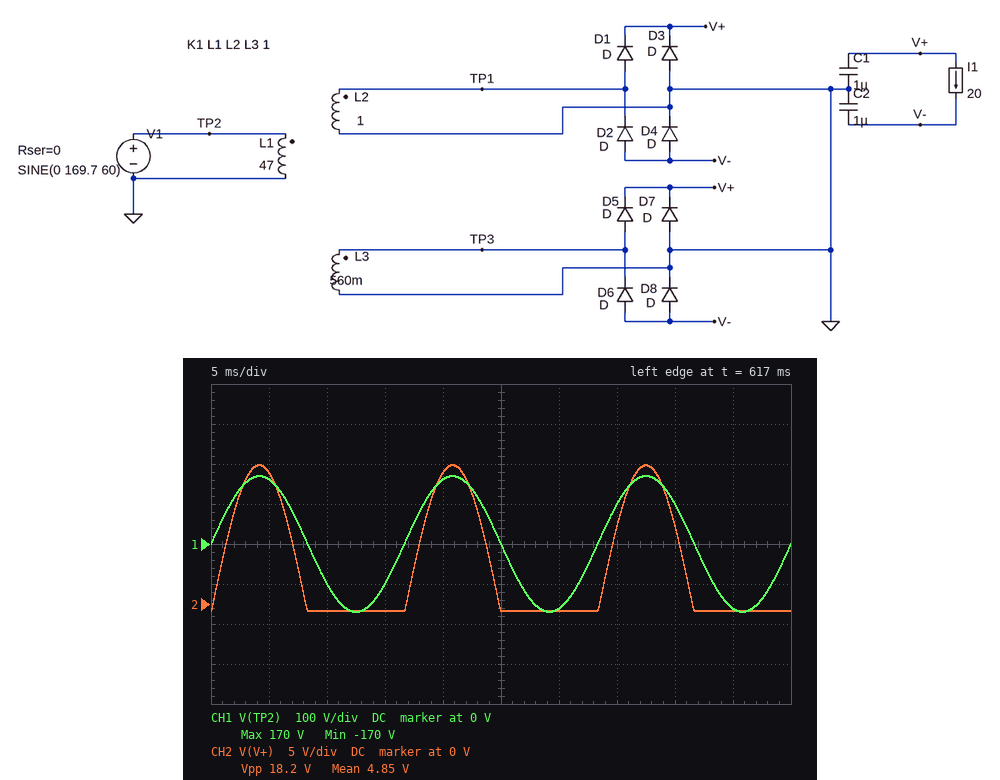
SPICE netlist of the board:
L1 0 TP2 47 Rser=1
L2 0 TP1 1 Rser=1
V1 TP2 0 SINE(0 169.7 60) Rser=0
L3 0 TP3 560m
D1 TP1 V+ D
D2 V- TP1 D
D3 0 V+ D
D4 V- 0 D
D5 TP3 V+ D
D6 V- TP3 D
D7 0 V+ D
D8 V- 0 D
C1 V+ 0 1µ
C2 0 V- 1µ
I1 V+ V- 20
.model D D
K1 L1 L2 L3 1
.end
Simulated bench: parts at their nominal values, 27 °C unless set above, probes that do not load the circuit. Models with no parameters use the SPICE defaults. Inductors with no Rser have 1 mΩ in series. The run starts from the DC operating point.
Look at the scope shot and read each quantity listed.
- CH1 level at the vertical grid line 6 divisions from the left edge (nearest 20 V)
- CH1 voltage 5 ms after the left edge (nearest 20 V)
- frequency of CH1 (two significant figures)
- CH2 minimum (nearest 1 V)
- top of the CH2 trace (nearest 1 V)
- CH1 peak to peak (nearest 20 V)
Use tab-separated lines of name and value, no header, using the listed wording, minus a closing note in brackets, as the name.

CH1 level at the vertical grid line 6 divisions from the left edge	-160 V
CH1 voltage 5 ms after the left edge	160 V
frequency of CH1	60 Hz
CH2 minimum	-1 V
top of the CH2 trace	17 V
CH1 peak to peak	340 V
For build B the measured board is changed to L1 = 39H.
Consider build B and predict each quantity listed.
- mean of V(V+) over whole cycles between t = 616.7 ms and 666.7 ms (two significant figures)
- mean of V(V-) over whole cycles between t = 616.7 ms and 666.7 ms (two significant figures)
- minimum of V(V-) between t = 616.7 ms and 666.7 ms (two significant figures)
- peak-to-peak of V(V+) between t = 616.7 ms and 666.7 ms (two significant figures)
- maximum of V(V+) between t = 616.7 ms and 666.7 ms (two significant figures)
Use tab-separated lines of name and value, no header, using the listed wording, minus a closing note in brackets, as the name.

mean of V(V+) over whole cycles between t = 616.7 ms and 666.7 ms	5.4 V
mean of V(V-) over whole cycles between t = 616.7 ms and 666.7 ms	-5.4 V
minimum of V(V-) between t = 616.7 ms and 666.7 ms	-19 V
peak-to-peak of V(V+) between t = 616.7 ms and 666.7 ms	20 V
maximum of V(V+) between t = 616.7 ms and 666.7 ms	19 V
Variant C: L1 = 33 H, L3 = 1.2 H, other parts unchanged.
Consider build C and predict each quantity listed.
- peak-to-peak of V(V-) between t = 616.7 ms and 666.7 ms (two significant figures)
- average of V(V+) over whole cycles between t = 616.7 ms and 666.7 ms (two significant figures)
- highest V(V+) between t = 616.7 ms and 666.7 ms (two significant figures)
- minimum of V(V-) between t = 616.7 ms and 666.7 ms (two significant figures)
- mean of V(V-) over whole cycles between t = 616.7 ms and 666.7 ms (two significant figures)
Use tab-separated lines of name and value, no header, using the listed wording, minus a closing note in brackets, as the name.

peak-to-peak of V(V-) between t = 616.7 ms and 666.7 ms	32 V
average of V(V+) over whole cycles between t = 616.7 ms and 666.7 ms	9.0 V
highest V(V+) between t = 616.7 ms and 666.7 ms	31 V
minimum of V(V-) between t = 616.7 ms and 666.7 ms	-31 V
mean of V(V-) over whole cycles between t = 616.7 ms and 666.7 ms	-9.0 V
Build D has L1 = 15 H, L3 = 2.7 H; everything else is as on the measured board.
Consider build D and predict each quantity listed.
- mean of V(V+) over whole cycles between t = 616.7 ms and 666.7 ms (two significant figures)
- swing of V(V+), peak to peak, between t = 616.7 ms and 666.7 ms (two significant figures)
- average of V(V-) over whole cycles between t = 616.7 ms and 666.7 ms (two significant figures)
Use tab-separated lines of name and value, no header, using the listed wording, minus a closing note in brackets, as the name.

mean of V(V+) over whole cycles between t = 616.7 ms and 666.7 ms	20 V
swing of V(V+), peak to peak, between t = 616.7 ms and 666.7 ms	68 V
average of V(V-) over whole cycles between t = 616.7 ms and 666.7 ms	-20 V
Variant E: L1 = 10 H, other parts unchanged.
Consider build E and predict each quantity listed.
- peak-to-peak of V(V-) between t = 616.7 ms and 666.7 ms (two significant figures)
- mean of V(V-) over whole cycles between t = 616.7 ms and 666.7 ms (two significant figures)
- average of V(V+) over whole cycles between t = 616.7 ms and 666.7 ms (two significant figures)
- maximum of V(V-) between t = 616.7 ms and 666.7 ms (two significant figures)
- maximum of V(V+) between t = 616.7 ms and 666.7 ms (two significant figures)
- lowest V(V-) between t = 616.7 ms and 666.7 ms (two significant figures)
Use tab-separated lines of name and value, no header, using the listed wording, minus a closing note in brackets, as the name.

peak-to-peak of V(V-) between t = 616.7 ms and 666.7 ms	39 V
mean of V(V-) over whole cycles between t = 616.7 ms and 666.7 ms	-11 V
average of V(V+) over whole cycles between t = 616.7 ms and 666.7 ms	11 V
maximum of V(V-) between t = 616.7 ms and 666.7 ms	890 mV
maximum of V(V+) between t = 616.7 ms and 666.7 ms	38 V
lowest V(V-) between t = 616.7 ms and 666.7 ms	-38 V
